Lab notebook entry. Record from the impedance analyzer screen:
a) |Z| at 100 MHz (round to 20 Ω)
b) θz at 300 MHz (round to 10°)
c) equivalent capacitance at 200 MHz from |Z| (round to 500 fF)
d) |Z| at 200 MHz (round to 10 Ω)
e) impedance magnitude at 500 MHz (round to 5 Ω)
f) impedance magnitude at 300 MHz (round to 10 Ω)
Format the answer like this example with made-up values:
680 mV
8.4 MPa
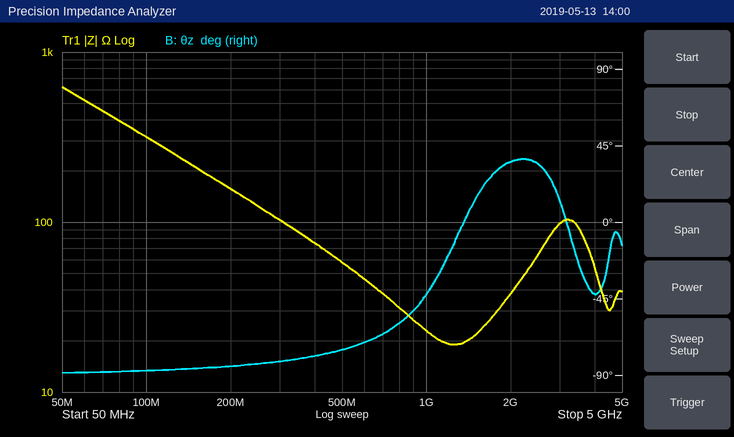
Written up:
320 Ω
-80°
5.0 pF
160 Ω
60 Ω
100 Ω
